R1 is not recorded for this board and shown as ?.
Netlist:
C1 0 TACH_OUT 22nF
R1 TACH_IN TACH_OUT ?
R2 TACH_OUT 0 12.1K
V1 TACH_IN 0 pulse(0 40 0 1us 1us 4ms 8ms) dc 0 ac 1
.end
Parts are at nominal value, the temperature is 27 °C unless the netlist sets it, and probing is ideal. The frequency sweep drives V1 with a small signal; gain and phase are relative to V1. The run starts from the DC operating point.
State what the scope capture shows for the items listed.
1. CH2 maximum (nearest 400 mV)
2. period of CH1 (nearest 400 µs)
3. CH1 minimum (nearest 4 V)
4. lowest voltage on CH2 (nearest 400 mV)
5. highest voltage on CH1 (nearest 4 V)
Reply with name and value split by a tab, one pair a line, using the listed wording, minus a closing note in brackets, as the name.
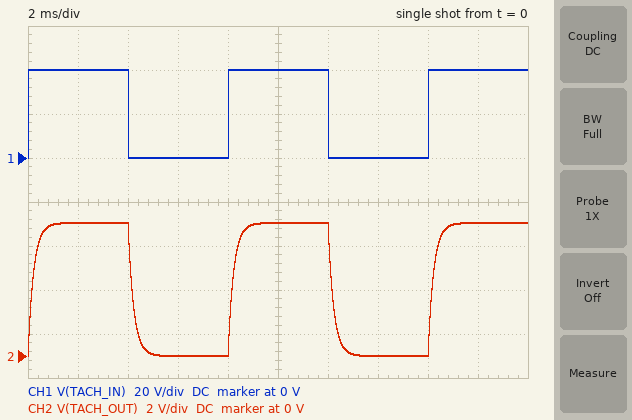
CH2 maximum	6.0 V
period of CH1	8.0 ms
CH1 minimum	0 V
lowest voltage on CH2	0 V
highest voltage on CH1	40 V
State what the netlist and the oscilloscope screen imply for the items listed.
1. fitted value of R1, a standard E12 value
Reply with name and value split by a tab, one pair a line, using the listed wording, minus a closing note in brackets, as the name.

fitted value of R1, a standard E12 value	68 kΩ
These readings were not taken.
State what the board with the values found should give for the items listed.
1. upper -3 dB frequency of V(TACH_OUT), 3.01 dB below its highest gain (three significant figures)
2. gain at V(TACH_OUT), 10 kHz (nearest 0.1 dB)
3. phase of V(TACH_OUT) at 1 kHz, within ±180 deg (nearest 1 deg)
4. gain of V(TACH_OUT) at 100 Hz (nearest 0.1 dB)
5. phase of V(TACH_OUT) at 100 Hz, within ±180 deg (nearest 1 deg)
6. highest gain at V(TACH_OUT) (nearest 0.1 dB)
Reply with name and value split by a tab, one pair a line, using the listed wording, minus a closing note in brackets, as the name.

upper -3 dB frequency of V(TACH_OUT), 3.01 dB below its highest gain	704 Hz
gain at V(TACH_OUT), 10 kHz	-39.5 dB
phase of V(TACH_OUT) at 1 kHz, within ±180 deg	-55 deg
gain of V(TACH_OUT) at 100 Hz	-16.5 dB
phase of V(TACH_OUT) at 100 Hz, within ±180 deg	-8 deg
highest gain at V(TACH_OUT)	-16.4 dB
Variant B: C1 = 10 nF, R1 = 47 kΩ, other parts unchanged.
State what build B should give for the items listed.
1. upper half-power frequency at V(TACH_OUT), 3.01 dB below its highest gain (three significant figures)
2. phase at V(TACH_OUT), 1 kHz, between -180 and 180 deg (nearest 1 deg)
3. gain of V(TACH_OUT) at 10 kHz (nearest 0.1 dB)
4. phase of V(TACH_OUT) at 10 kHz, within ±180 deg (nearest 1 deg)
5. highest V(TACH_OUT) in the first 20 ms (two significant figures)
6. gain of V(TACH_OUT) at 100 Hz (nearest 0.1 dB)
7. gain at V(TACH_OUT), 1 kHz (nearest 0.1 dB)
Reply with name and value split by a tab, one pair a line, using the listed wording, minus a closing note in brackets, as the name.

upper half-power frequency at V(TACH_OUT), 3.01 dB below its highest gain	1.65 kHz
phase at V(TACH_OUT), 1 kHz, between -180 and 180 deg	-31 deg
gain of V(TACH_OUT) at 10 kHz	-29.5 dB
phase of V(TACH_OUT) at 10 kHz, within ±180 deg	-81 deg
highest V(TACH_OUT) in the first 20 ms	8.2 V
gain of V(TACH_OUT) at 100 Hz	-13.8 dB
gain at V(TACH_OUT), 1 kHz	-15.1 dB
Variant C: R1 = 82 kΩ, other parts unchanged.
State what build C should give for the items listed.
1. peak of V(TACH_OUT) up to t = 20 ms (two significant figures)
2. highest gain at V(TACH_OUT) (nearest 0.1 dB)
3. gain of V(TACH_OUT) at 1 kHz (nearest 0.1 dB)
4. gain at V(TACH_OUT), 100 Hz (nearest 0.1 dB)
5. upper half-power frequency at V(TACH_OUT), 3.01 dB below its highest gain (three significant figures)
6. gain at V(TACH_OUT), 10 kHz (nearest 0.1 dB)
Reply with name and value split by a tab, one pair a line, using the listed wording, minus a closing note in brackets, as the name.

peak of V(TACH_OUT) up to t = 20 ms	5.1 V
highest gain at V(TACH_OUT)	-17.8 dB
gain of V(TACH_OUT) at 1 kHz	-22.8 dB
gain at V(TACH_OUT), 100 Hz	-17.9 dB
upper half-power frequency at V(TACH_OUT), 3.01 dB below its highest gain	686 Hz
gain at V(TACH_OUT), 10 kHz	-41.1 dB
